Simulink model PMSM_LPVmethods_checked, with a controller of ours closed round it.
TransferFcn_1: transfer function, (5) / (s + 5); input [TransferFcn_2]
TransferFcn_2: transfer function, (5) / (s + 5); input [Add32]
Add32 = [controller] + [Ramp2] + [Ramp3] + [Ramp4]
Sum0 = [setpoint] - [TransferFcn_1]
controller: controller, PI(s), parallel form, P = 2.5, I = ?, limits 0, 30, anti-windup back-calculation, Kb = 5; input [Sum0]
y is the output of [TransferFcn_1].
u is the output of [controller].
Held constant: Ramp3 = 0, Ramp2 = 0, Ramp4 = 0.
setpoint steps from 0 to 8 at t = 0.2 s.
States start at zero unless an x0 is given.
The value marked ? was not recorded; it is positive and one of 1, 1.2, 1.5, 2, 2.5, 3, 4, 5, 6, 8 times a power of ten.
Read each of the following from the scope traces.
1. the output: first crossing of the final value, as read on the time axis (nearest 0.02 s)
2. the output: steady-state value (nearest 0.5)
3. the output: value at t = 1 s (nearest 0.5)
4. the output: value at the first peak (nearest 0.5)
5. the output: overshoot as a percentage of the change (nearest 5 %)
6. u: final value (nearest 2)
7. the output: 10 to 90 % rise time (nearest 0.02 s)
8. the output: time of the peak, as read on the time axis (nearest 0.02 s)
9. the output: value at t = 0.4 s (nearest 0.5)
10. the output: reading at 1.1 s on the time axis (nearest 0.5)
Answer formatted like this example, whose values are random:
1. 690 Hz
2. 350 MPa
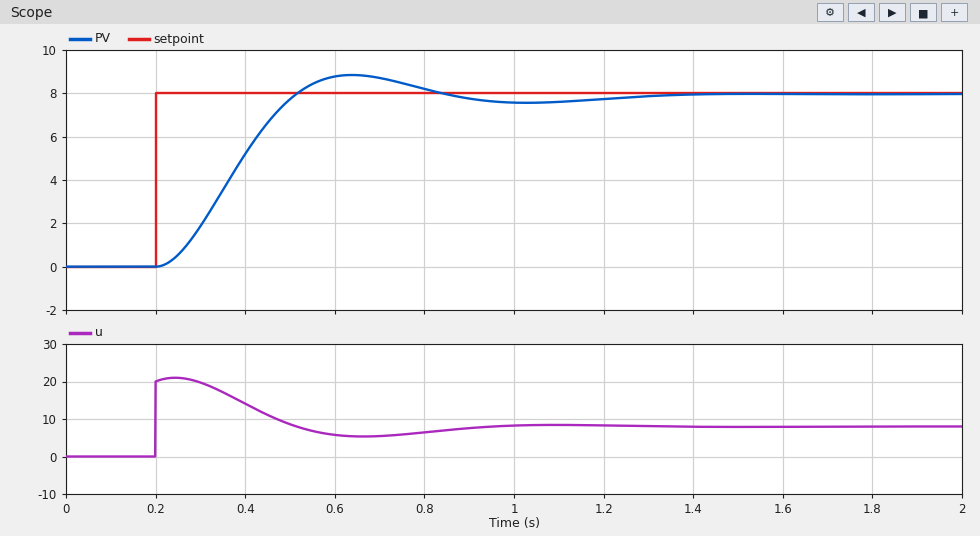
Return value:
1. 0.52 s
2. 8.0
3. 7.5
4. 9.0
5. 10 %
6. 8
7. 0.22 s
8. 0.64 s
9. 5.0
10. 7.5
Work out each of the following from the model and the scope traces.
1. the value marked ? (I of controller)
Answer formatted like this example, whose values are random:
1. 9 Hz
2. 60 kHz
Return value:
1. 6
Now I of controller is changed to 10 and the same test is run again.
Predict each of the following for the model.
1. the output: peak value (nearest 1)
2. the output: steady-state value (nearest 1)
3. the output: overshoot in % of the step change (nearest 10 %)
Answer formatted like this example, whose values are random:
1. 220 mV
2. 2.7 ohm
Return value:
1. 10
2. 8
3. 30 %
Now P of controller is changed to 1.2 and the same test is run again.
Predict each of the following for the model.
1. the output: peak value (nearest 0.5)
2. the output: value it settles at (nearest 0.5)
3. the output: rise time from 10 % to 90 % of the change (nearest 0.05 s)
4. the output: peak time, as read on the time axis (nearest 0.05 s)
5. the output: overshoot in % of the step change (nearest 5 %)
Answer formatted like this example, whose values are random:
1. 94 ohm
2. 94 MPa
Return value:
1. 9.5
2. 8.0
3. 0.30 s
4. 0.85 s
5. 20 %
